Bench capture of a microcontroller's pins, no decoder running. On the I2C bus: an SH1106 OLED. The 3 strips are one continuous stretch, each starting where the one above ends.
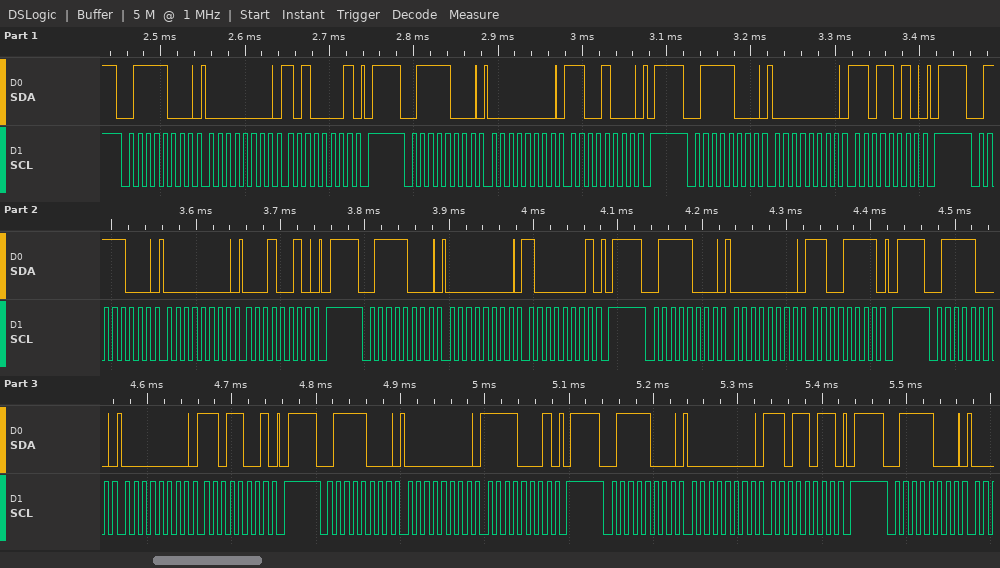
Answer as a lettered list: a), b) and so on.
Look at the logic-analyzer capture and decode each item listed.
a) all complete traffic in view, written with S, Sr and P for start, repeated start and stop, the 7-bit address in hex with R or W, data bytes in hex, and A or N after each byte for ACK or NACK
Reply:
a) S 3CW A 00 A A1 A P S 3CW A 00 A C8 A P S 3CW A 00 A DA A P S 3CW A 00 A 12 A P S 3CW A 00 A 81 A P S 3CW A 00 A CF A P S 3CW A 00 A D9 A P S 3CW A 00 A F1 A P S 3CW A 00 A DB A P S 3CW A
